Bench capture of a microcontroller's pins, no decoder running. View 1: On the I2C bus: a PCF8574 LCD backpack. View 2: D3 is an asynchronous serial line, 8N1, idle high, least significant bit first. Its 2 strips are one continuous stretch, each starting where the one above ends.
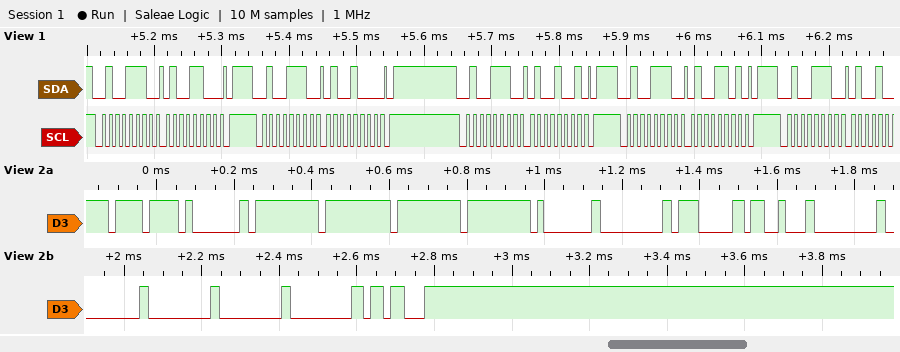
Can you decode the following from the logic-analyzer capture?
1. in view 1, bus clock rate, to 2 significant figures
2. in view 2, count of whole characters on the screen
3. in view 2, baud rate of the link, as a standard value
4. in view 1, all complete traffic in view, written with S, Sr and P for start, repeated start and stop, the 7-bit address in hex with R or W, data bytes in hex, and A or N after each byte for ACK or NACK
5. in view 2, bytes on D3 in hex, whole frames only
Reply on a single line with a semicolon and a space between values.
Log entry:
100 kHz; 16; 57600 baud; S 27W A 4C A P S 27W A 48 A P S 27W A 49 A P S 27W A 4D A P S 27W A; 0xEF 0x01 0xFF 0xFF 0xFF 0xFF 0x01 0x00 0x07 0x13 0x00 0x00 0x00 0x00 0x00 0x1B
